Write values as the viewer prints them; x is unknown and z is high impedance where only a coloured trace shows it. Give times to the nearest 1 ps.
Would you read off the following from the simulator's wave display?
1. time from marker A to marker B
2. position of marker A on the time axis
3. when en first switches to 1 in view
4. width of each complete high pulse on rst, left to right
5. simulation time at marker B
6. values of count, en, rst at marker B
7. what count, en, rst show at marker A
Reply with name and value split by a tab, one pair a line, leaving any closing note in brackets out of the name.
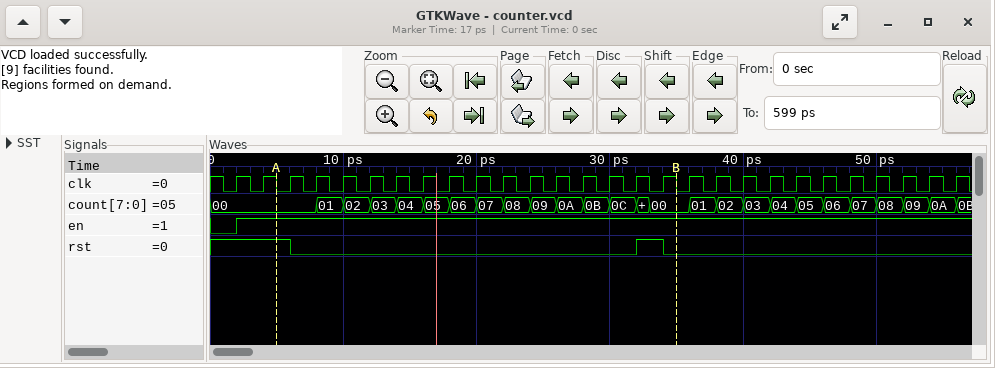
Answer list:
time from marker A to marker B	30 ps
position of marker A on the time axis	5 ps
when en first switches to 1 in view	2 ps
width of each complete high pulse on rst, left to right	2 ps
simulation time at marker B	35 ps
values of count, en, rst at marker B	count=00, en=1, rst=0
what count, en, rst show at marker A	count=00, en=1, rst=1
